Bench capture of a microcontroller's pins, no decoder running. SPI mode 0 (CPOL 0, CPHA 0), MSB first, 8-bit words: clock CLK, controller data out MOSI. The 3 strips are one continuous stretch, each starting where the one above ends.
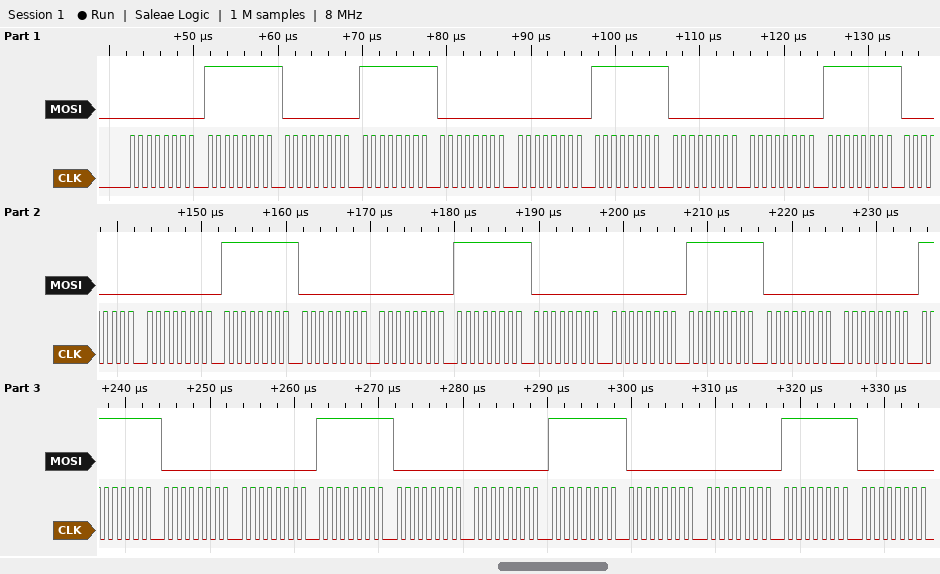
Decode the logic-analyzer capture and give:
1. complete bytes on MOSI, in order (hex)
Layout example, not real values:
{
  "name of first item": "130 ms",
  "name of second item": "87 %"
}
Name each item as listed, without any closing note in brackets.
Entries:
{
  "complete bytes on MOSI, in order": "00 FF 00 FF 00 00 FF 00 00 FF 00 00 FF 00 00 FF 00 00 FF 00 00 FF 00 00 FF 00 00 FF 00 00 FF 00"
}
